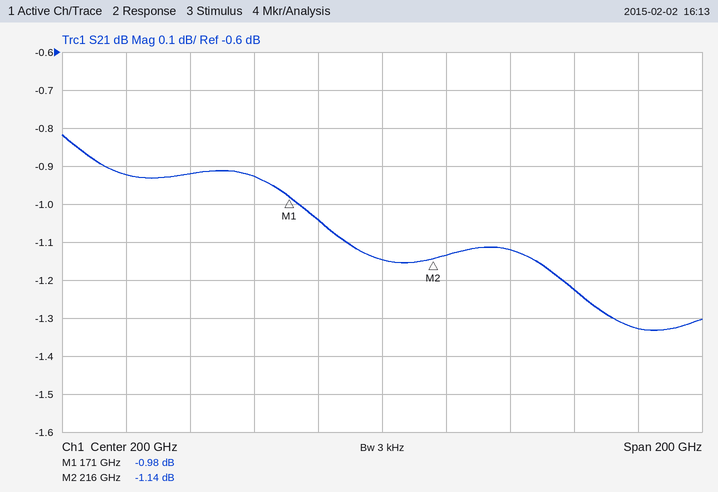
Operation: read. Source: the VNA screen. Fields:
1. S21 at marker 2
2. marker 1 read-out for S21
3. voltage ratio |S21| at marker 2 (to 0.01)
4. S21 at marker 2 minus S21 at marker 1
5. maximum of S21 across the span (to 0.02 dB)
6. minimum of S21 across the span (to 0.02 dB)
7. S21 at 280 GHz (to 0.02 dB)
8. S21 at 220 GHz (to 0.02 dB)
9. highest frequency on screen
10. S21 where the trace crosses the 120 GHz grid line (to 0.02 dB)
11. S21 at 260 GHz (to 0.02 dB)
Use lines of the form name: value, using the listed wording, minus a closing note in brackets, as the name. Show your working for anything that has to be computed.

S21 at marker 2: -1.14 dB
marker 1 read-out for S21: -0.98 dB
voltage ratio |S21| at marker 2: 10^(-1.14/20) ≈ 0.88
S21 at marker 2 minus S21 at marker 1: -1.14 − (-0.98) = -0.16 dB
maximum of S21 across the span: -0.82 dB
minimum of S21 across the span: -1.34 dB
S21 at 280 GHz: -1.32 dB
S21 at 220 GHz: -1.14 dB
highest frequency on screen: 300 GHz
S21 where the trace crosses the 120 GHz grid line: -0.92 dB
S21 at 260 GHz: -1.22 dB
